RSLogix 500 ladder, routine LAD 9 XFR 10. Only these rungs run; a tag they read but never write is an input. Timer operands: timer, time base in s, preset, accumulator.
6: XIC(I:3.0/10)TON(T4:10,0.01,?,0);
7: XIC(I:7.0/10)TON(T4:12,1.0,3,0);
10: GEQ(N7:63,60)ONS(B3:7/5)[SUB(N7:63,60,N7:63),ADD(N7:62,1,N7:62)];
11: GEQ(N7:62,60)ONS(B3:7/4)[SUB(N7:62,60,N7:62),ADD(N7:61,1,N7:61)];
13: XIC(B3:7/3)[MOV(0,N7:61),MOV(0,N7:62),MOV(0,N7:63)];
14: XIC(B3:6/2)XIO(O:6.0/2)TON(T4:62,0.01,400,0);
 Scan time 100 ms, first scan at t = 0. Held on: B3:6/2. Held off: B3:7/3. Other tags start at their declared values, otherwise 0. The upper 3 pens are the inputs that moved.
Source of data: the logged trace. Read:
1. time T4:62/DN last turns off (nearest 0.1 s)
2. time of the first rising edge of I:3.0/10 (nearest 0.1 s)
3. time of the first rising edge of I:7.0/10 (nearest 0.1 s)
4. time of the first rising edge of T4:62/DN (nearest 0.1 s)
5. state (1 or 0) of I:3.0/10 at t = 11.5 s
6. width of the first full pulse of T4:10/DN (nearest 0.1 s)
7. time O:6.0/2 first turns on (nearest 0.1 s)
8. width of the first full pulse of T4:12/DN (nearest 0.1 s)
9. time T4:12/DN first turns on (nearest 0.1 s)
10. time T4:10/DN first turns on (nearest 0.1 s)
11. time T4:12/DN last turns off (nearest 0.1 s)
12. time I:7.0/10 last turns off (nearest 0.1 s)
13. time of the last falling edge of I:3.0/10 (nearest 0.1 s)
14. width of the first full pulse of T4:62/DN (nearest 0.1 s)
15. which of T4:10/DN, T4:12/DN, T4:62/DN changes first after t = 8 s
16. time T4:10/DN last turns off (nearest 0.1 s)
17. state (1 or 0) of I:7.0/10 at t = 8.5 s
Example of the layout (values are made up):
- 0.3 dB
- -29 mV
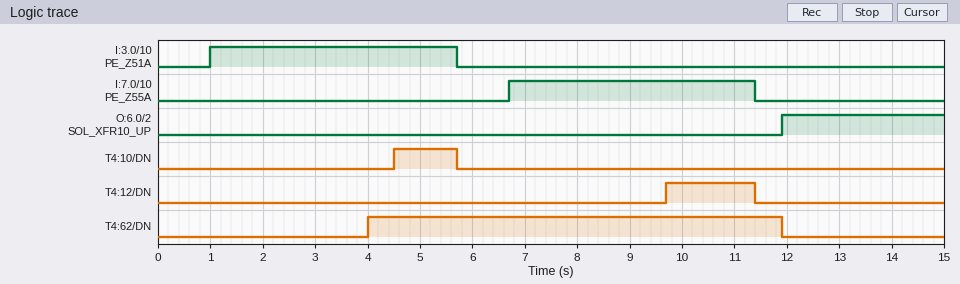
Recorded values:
- 11.9 s
- 1.0 s
- 6.7 s
- 4.0 s
- 0
- 1.2 s
- 11.9 s
- 1.7 s
- 9.7 s
- 4.5 s
- 11.4 s
- 11.4 s
- 5.7 s
- 7.9 s
- T4:12/DN
- 5.7 s
- 1
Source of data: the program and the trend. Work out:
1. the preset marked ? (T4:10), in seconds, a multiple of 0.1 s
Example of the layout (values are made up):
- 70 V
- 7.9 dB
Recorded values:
- 3.5 s
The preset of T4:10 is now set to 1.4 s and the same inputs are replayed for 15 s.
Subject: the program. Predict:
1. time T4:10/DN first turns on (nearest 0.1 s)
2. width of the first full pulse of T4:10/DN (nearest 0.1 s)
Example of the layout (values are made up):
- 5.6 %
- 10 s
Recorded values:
- 2.4 s
- 3.3 s
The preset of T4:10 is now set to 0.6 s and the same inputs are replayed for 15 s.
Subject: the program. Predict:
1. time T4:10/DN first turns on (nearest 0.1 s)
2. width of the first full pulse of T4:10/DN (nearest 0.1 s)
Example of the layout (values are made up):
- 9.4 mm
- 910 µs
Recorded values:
- 1.6 s
- 4.1 s
